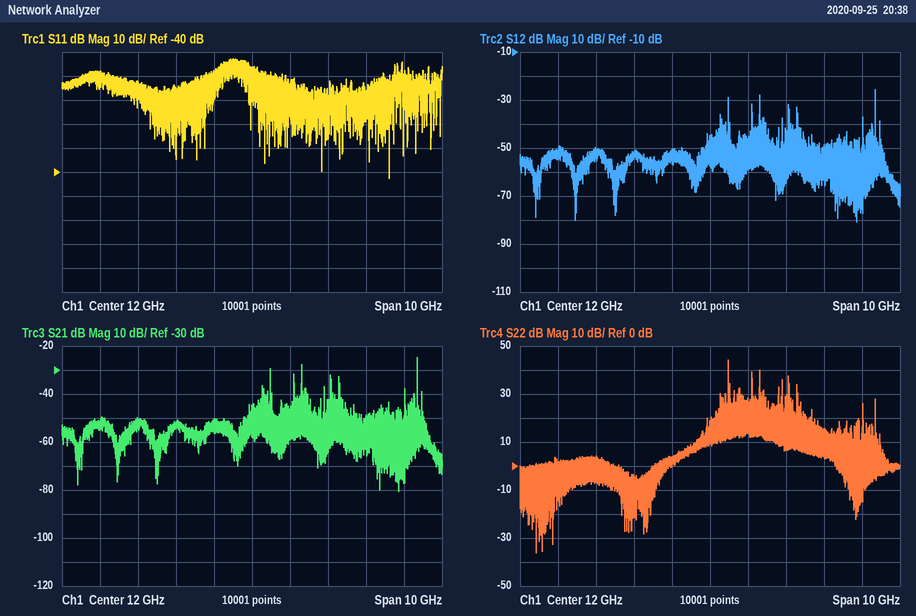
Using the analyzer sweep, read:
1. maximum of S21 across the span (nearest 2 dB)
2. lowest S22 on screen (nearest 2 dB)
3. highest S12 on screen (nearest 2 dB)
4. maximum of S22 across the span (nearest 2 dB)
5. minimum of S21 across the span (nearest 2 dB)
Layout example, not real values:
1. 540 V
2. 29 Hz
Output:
1. -24 dB
2. -36 dB
3. -26 dB
4. 44 dB
5. -80 dB
